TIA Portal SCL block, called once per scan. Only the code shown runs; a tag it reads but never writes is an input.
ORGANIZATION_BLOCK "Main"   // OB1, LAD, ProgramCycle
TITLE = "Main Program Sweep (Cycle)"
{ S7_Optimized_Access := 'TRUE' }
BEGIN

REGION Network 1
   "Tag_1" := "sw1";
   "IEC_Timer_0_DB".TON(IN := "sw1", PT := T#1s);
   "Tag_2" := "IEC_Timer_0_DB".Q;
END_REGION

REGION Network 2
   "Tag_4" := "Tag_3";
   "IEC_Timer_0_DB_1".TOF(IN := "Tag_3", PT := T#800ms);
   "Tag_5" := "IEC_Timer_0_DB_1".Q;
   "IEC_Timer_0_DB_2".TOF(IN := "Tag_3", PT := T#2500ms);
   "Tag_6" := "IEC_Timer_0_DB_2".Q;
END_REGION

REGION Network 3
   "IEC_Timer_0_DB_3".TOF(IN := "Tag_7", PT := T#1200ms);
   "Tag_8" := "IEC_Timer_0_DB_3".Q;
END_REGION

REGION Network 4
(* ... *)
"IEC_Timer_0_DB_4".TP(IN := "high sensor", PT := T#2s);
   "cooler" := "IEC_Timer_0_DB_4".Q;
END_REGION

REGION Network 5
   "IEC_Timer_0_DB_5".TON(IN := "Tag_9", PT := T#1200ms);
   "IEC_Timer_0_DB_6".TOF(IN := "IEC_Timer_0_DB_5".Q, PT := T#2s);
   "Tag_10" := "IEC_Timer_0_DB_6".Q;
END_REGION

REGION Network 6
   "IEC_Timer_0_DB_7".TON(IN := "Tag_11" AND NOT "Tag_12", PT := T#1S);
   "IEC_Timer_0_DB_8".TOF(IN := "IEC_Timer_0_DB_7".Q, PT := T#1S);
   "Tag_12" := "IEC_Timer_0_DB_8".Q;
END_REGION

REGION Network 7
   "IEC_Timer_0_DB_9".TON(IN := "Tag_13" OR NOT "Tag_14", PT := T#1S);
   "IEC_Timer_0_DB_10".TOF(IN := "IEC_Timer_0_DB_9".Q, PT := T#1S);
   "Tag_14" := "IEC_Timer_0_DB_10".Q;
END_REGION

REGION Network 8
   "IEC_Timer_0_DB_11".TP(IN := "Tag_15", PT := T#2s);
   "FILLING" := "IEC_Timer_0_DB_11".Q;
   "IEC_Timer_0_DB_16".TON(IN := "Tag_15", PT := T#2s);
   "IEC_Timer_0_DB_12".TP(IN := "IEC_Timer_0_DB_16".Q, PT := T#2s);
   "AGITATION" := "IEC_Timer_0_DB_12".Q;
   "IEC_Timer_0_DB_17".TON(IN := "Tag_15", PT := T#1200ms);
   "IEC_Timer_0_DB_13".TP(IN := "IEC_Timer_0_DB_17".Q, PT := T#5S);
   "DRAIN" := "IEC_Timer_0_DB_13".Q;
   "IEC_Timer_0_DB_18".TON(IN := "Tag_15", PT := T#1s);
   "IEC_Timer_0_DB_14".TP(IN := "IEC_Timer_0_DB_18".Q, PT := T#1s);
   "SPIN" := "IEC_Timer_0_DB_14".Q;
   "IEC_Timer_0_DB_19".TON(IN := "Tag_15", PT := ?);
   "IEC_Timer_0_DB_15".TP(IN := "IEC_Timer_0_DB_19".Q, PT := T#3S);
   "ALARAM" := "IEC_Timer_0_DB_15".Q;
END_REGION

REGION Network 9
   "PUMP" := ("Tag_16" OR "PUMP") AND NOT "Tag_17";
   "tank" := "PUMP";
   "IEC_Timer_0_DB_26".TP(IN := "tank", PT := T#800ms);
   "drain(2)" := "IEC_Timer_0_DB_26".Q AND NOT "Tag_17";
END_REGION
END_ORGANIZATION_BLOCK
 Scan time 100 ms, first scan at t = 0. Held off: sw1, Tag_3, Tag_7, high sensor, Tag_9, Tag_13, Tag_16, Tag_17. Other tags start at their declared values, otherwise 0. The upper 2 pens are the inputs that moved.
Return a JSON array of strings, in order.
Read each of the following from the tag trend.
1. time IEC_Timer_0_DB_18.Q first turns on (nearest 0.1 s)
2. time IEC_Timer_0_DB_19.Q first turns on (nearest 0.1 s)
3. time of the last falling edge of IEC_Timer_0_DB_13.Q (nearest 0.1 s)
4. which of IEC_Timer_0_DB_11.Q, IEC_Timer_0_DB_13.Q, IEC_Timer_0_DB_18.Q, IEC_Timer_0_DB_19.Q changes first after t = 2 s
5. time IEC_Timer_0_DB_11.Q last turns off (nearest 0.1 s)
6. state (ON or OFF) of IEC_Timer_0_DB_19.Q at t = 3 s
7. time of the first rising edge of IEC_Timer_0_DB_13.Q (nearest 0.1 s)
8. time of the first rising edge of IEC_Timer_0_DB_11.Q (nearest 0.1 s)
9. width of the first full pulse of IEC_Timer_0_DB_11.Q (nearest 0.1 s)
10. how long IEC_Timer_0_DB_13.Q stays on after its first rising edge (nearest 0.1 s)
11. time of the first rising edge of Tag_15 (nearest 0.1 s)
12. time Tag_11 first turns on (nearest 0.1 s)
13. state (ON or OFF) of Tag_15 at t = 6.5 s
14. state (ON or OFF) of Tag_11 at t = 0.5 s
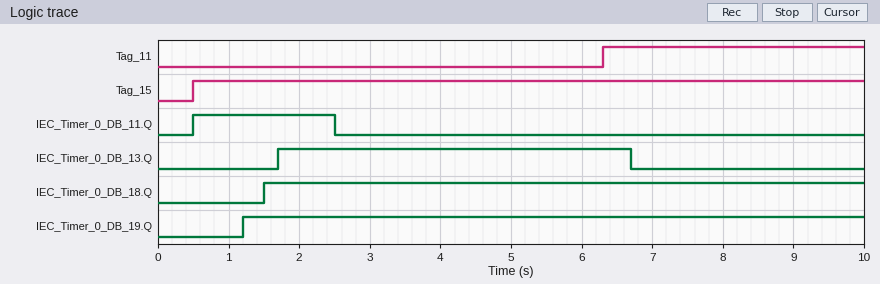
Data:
["1.5 s", "1.2 s", "6.7 s", "IEC_Timer_0_DB_11.Q", "2.5 s", "ON", "1.7 s", "0.5 s", "2.0 s", "5.0 s", "0.5 s", "6.3 s", "ON", "OFF"]
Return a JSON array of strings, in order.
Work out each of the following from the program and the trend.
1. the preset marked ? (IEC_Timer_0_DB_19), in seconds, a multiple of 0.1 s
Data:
["0.7 s"]
